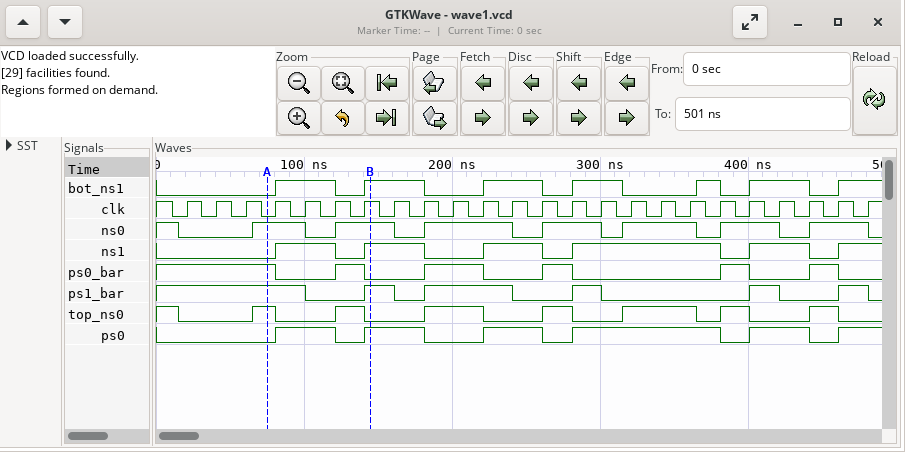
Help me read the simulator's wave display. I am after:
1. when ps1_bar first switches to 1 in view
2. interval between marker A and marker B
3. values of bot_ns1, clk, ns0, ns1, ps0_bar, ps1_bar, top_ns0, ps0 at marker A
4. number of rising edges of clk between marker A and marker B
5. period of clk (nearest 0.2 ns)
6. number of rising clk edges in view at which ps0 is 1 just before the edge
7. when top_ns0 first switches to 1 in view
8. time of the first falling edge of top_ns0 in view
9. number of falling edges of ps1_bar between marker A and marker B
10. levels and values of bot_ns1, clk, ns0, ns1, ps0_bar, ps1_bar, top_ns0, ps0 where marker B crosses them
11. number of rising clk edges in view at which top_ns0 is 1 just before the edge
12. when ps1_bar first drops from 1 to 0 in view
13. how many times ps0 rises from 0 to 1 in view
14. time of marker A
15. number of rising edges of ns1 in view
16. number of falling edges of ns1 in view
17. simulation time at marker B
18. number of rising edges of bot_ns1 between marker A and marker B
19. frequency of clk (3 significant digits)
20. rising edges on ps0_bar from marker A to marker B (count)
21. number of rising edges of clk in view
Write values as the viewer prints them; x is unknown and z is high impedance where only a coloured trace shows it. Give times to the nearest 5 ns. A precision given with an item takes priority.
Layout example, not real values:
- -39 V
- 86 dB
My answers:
- 140 ns
- 70 ns
- bot_ns1=0, clk=0, ns0=1, ns1=0, ps0_bar=1, ps1_bar=1, top_ns0=1, ps0=0
- 4
- 20 ns
- 14
- 65 ns
- 15 ns
- 1
- bot_ns1=1, clk=1, ns0=1, ns1=1, ps0_bar=0, ps1_bar=1, top_ns0=0, ps0=1
- 10
- 100 ns
- 6
- 75 ns
- 6
- 5
- 145 ns
- 2
- 50.0 MHz
- 1
- 24
